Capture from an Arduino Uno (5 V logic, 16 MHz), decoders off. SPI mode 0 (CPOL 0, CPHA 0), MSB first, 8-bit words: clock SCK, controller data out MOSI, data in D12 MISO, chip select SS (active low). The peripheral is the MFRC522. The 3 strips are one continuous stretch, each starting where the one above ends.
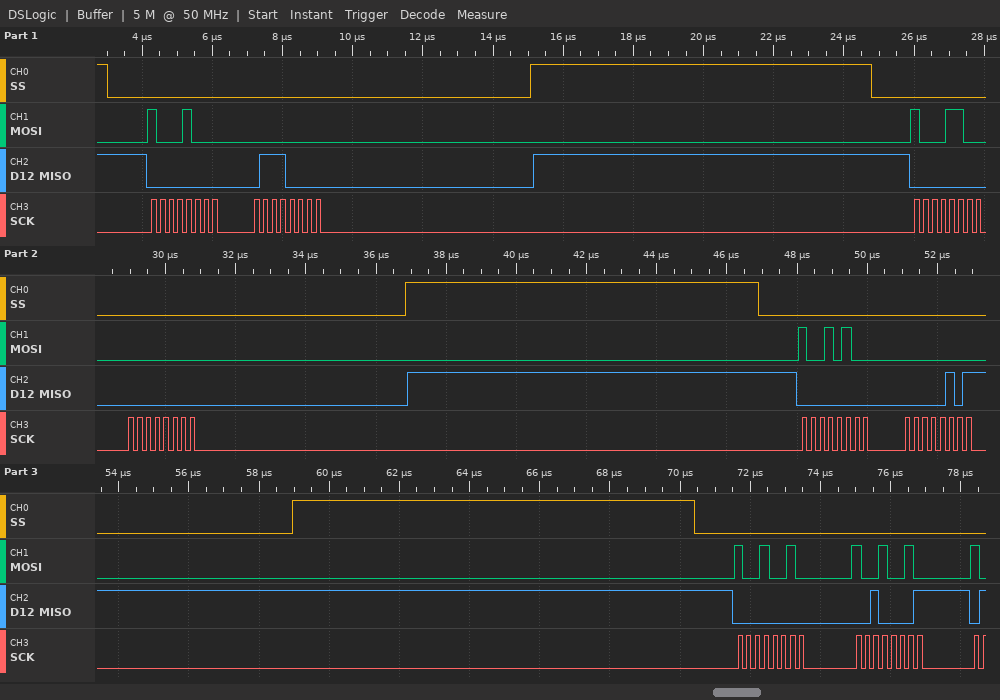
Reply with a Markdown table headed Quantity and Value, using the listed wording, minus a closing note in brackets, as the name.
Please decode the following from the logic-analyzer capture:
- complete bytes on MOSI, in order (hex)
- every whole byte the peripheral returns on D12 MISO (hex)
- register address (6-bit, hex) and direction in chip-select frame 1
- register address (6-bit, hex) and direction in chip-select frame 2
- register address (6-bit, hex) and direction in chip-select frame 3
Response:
| Quantity | Value |
|---|---|
| complete bytes on MOSI, in order | 88 00 8C 00 94 00 92 92 |
| every whole byte the peripheral returns on D12 MISO | 00 70 00 00 00 05 00 21 |
| register address (6-bit, hex) and direction in chip-select frame 1 | 0x04 read |
| register address (6-bit, hex) and direction in chip-select frame 2 | 0x06 read |
| register address (6-bit, hex) and direction in chip-select frame 3 | 0x0A read |
